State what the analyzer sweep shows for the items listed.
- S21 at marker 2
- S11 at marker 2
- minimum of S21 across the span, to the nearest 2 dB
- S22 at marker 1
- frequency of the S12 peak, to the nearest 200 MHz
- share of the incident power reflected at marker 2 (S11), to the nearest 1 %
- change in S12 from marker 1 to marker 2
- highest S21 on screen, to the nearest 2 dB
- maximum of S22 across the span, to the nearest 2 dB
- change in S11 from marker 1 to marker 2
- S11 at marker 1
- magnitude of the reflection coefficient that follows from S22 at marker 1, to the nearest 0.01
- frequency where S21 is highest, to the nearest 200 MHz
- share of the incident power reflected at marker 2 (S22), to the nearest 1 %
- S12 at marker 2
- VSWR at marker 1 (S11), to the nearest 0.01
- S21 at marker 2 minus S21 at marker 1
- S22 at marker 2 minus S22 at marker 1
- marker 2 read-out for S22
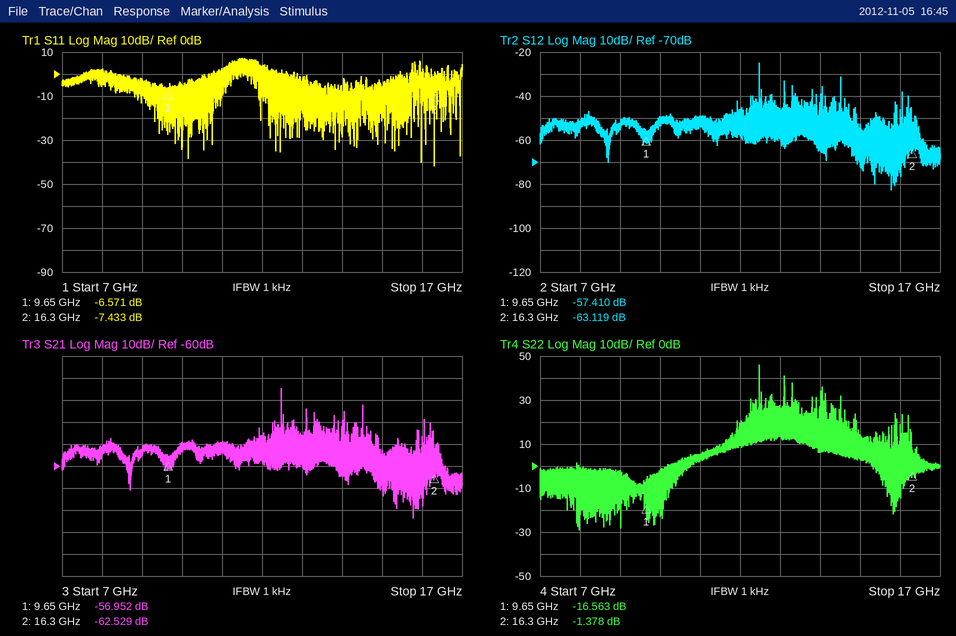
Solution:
-62.529 dB
-7.433 dB
-84 dB
-16.563 dB
12.4 GHz
18 %
-5.709 dB
-24 dB
46 dB
-0.862 dB
-6.571 dB
0.15
12.4 GHz
73 %
-63.119 dB
2.77
-5.577 dB
15.185 dB
-1.378 dB
